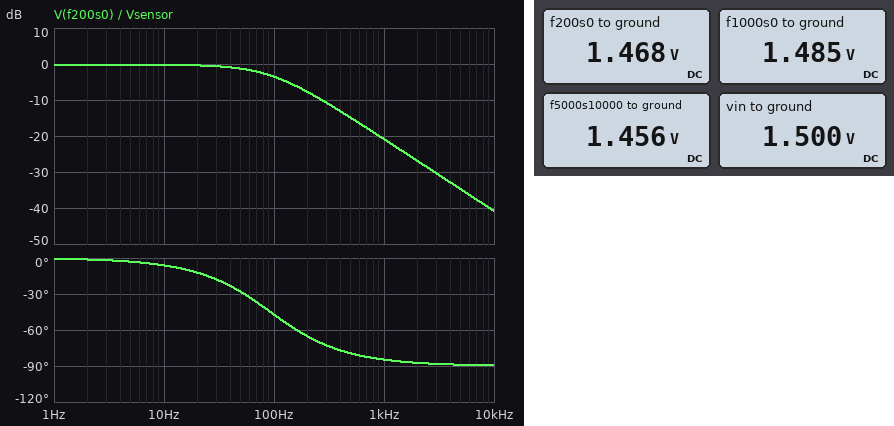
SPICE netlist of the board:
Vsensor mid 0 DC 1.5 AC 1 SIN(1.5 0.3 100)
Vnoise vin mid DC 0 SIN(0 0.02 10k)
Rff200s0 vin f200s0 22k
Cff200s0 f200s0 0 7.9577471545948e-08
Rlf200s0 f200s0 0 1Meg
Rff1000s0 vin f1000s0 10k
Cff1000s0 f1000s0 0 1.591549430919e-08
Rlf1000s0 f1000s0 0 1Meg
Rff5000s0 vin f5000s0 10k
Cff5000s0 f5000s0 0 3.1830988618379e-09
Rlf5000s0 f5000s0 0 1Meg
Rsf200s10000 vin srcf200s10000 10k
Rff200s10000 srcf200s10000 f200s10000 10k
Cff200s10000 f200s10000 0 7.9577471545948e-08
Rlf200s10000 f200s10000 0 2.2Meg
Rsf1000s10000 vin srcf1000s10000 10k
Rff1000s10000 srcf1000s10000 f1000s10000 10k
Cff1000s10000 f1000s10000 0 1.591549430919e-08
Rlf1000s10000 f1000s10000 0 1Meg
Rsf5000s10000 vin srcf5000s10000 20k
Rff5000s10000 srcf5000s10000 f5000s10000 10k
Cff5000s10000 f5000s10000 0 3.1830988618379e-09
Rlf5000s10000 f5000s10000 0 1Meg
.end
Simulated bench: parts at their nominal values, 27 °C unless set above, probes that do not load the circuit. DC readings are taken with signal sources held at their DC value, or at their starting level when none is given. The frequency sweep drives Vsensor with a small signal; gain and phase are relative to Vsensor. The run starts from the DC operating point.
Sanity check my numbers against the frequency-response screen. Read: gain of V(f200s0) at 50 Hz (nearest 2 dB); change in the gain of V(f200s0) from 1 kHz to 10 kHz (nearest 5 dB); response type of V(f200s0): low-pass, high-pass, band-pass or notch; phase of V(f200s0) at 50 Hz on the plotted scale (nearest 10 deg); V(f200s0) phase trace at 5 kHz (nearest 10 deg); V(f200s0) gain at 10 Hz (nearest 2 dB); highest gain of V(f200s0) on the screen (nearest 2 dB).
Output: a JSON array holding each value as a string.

["-2 dB", "-20 dB", "low-pass", "-30 deg", "-90 deg", "0 dB", "0 dB"]
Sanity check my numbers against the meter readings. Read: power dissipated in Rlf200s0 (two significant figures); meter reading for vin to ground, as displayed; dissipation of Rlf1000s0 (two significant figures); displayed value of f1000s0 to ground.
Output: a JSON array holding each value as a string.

["2.2 µW", "1.500 V", "2.2 µW", "1.485 V"]
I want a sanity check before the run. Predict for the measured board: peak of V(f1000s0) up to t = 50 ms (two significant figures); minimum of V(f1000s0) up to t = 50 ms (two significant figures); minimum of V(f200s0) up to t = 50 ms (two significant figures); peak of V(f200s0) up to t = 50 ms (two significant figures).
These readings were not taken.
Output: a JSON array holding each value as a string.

["1.8 V", "1.2 V", "1.3 V", "1.7 V"]
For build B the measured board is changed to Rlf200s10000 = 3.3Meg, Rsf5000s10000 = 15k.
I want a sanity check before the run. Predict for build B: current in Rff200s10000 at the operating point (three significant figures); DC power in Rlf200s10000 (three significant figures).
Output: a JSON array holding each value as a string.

["452 nA", "674 nW"]
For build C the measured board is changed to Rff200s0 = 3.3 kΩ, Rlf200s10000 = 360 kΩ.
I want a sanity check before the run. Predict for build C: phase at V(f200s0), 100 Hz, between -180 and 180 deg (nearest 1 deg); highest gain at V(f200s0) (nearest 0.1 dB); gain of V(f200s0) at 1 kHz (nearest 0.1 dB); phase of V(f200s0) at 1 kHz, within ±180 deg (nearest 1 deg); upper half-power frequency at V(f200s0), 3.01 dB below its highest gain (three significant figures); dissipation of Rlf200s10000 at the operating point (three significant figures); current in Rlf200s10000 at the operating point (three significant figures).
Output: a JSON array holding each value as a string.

["-9 deg", "0 dB", "-5.7 dB", "-59 deg", "608 Hz", "5.61 µW", "3.95 µA"]
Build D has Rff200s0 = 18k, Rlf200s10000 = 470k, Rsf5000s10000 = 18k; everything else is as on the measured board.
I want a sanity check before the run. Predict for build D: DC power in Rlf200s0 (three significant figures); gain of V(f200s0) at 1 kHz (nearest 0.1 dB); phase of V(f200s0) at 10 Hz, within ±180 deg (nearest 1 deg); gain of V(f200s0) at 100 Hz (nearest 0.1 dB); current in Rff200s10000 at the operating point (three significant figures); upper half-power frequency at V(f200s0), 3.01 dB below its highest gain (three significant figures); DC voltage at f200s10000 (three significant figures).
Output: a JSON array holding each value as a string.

["2.17 µW", "-19.1 dB", "-5 deg", "-2.7 dB", "3.06 µA", "113 Hz", "1.44 V"]
